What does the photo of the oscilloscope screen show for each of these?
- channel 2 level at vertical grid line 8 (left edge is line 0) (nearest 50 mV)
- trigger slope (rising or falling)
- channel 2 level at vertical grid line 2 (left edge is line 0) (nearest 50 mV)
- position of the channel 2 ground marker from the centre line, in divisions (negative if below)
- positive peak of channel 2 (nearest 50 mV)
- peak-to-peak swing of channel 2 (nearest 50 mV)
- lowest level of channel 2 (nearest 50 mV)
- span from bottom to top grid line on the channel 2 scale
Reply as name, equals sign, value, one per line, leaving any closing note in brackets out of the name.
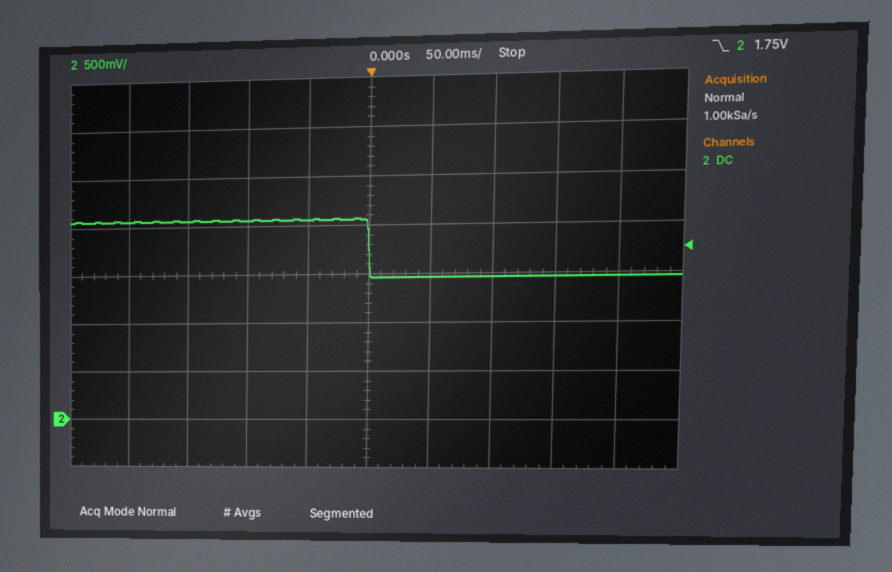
channel 2 level at vertical grid line 8 (left edge is line 0) = 1.45 V
trigger slope = falling
channel 2 level at vertical grid line 2 (left edge is line 0) = 2.05 V
position of the channel 2 ground marker from the centre line, in divisions = -3.0 div
positive peak of channel 2 = 2.05 V
peak-to-peak swing of channel 2 = 600 mV
lowest level of channel 2 = 1.45 V
span from bottom to top grid line on the channel 2 scale = 4 V
